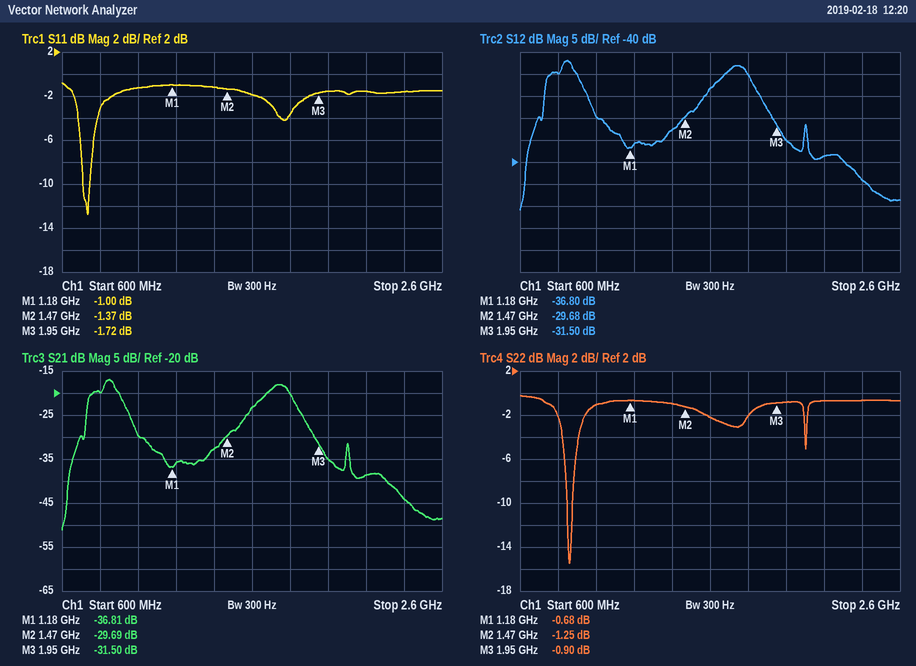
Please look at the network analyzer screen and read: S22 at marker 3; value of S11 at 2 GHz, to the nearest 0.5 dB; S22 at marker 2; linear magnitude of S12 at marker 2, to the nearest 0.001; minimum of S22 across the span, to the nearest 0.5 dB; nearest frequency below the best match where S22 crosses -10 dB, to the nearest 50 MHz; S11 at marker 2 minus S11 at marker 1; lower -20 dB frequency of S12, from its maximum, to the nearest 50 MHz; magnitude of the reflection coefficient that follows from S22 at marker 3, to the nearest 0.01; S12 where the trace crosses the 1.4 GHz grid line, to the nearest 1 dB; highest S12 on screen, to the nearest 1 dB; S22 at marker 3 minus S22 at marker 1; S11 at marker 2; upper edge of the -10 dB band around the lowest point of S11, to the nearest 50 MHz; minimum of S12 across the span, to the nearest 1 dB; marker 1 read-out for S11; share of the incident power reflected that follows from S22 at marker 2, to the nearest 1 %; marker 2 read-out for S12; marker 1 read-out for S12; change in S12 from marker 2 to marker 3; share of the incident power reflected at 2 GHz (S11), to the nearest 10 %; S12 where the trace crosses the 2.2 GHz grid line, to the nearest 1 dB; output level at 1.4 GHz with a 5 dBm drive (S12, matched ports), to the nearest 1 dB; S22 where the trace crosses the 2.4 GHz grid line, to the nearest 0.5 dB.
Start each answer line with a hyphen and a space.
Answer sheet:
- -0.90 dB
- -1.5 dB
- -1.25 dB
- 0.033
- -15.5 dB
- 850 MHz
- -0.37 dB
- 650 MHz
- 0.90
- -33 dB
- -17 dB
- -0.22 dB
- -1.37 dB
- 750 MHz
- -51 dB
- -1.00 dB
- 75 %
- -29.68 dB
- -36.80 dB
- -1.82 dB
- 70 %
- -39 dB
- -28 dBm
- -0.5 dB
